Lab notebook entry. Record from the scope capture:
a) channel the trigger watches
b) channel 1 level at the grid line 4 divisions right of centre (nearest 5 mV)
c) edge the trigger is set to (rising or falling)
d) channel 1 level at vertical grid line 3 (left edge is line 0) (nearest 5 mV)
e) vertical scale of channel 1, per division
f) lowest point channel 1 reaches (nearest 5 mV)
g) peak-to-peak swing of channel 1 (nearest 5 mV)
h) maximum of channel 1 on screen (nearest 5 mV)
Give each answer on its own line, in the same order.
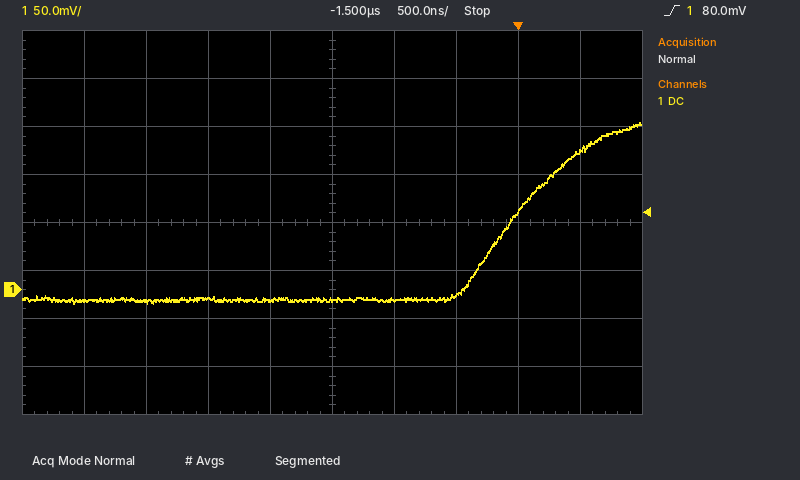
channel 1
145 mV
rising
-10 mV
50 mV
-15 mV
190 mV
175 mV
